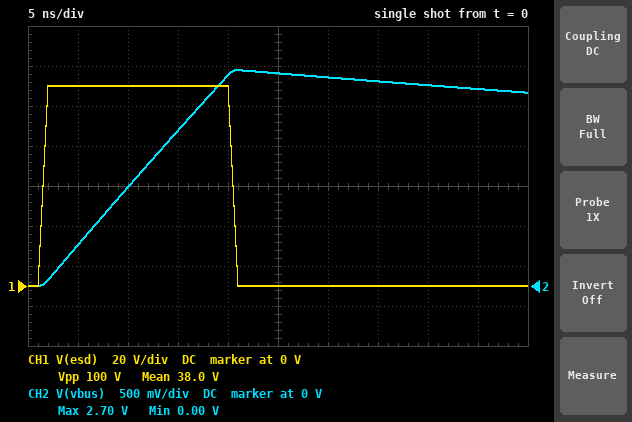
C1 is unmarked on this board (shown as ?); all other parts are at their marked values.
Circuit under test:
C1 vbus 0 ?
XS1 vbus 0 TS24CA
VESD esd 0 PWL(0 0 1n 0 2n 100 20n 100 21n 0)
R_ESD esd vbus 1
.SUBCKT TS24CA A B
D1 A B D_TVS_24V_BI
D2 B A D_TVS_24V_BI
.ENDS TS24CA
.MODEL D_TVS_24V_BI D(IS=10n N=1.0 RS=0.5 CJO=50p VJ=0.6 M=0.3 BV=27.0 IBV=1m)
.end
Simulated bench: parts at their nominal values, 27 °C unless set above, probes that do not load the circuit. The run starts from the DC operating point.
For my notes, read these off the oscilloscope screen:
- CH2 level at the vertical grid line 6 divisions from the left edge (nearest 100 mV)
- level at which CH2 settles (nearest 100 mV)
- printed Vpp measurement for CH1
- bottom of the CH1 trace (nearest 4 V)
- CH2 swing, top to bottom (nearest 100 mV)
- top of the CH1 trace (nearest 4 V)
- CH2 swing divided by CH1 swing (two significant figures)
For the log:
2.6 V
2.4 V
100 V
0 V
2.7 V
100 V
0.027
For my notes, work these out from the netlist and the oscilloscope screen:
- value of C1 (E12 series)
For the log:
680 nF
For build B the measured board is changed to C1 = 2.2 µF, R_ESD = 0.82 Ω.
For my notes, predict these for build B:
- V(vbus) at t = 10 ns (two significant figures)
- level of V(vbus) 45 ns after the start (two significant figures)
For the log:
470 mV
1.0 V
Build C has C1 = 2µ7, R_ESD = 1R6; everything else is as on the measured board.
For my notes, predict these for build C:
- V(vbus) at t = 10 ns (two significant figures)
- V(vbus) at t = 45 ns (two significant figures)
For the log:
200 mV
440 mV
